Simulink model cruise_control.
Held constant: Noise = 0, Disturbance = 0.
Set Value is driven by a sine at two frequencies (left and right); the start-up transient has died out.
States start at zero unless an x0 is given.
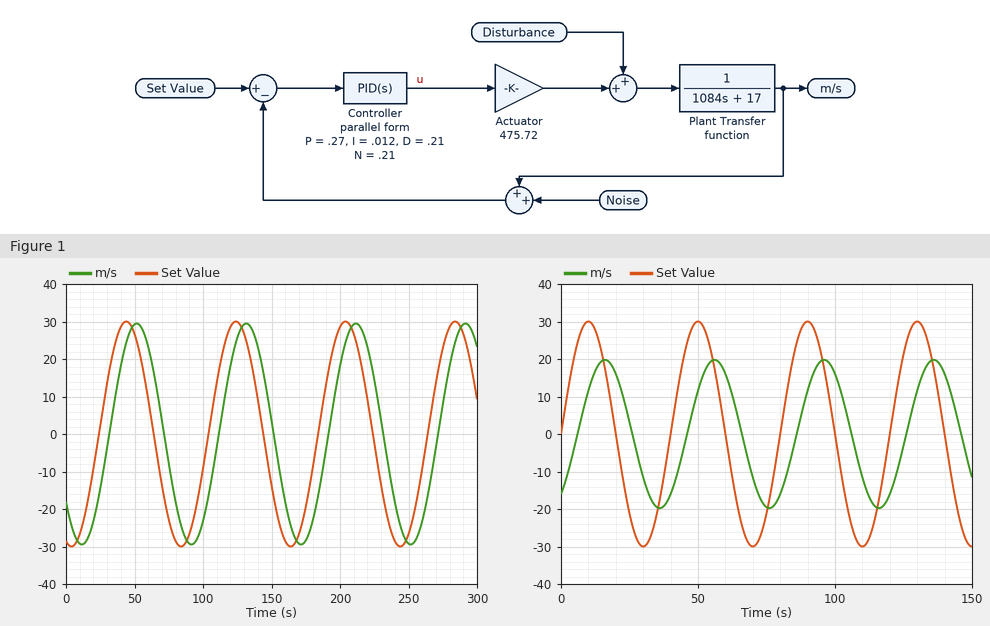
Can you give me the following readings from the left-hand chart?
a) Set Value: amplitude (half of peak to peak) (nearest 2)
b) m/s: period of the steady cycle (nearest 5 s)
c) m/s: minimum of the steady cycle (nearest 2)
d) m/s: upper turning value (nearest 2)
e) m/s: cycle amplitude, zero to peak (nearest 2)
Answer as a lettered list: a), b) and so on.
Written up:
a) 30
b) 80 s
c) -30
d) 30
e) 30
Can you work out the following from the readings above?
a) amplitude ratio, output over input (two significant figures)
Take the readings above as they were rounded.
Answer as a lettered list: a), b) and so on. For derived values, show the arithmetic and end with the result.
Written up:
a) 30 / 30 = 1.0
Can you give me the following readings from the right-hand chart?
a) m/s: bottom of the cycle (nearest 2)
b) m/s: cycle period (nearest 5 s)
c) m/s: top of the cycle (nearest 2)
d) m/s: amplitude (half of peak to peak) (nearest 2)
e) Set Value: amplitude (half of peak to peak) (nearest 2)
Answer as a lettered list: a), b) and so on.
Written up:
a) -20
b) 40 s
c) 20
d) 20
e) 30
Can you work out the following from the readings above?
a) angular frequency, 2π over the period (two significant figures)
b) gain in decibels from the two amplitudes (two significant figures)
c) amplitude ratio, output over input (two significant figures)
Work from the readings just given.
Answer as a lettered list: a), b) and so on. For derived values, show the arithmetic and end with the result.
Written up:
a) 2π / 40 = 0.16 rad/s
b) 20 log10(20 / 30) = -3.5 dB
c) 20 / 30 = 0.67
